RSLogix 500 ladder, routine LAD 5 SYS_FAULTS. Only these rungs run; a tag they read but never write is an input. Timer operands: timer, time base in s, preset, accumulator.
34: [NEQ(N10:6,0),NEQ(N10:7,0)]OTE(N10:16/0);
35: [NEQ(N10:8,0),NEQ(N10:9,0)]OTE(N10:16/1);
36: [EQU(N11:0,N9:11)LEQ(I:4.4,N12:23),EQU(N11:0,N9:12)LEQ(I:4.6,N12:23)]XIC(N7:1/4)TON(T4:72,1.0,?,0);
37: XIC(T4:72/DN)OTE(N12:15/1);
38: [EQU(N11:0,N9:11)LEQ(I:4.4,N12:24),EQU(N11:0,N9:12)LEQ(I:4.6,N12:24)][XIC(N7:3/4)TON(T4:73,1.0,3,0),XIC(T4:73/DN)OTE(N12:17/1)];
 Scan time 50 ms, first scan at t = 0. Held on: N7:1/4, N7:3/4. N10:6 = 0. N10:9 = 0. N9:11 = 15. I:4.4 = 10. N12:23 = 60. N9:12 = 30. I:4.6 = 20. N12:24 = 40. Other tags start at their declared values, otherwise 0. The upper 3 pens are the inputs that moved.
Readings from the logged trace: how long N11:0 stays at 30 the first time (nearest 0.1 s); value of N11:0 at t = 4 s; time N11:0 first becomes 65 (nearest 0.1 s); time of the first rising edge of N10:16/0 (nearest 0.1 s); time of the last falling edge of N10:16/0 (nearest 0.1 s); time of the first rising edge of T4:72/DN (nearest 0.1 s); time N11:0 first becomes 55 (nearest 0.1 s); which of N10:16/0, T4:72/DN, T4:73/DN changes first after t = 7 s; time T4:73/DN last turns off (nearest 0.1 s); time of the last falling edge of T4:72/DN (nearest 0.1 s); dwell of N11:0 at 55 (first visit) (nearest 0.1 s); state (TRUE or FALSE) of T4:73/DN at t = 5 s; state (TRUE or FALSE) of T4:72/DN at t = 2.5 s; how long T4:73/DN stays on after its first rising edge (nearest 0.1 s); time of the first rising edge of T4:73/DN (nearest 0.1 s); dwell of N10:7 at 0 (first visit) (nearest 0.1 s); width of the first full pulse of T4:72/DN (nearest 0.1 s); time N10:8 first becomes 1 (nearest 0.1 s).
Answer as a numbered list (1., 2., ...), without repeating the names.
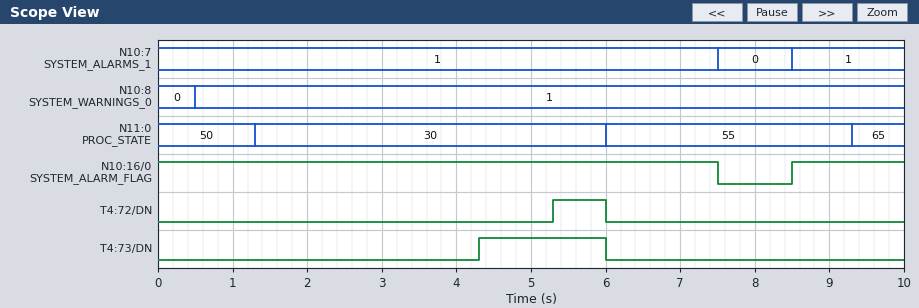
1. 4.7 s
2. 30
3. 9.3 s
4. 8.5 s
5. 7.5 s
6. 5.3 s
7. 6.0 s
8. N10:16/0
9. 6.0 s
10. 6.0 s
11. 3.3 s
12. TRUE
13. FALSE
14. 1.7 s
15. 4.3 s
16. 1.0 s
17. 0.7 s
18. 0.5 s
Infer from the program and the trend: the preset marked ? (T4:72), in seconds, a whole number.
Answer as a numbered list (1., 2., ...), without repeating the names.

1. 4 s
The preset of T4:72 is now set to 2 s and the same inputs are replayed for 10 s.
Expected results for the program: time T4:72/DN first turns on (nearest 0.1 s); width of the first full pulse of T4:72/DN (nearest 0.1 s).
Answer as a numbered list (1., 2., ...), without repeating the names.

1. 3.3 s
2. 2.7 s
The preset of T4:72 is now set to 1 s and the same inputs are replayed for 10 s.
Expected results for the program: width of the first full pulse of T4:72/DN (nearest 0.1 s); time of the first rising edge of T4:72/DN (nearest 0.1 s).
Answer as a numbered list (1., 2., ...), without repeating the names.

1. 3.7 s
2. 2.3 s
